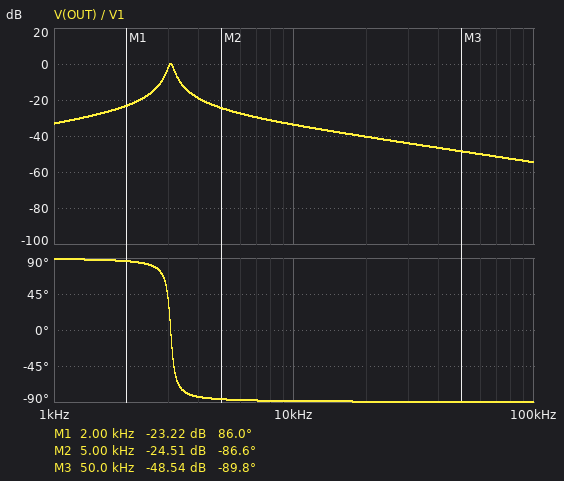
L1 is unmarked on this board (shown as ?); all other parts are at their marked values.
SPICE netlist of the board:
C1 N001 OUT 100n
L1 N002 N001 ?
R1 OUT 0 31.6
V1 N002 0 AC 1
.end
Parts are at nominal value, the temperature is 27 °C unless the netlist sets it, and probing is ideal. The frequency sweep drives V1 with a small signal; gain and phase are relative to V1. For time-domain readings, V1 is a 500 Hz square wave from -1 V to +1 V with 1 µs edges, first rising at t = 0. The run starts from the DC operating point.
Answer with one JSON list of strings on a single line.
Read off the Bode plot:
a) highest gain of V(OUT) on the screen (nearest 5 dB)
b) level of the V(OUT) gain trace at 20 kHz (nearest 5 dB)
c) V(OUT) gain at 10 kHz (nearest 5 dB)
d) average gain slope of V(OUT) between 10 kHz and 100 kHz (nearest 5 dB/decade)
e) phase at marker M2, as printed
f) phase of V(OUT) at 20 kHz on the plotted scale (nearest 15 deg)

["0 dB", "-40 dB", "-35 dB", "-20 dB/decade", "-86.6 deg", "-90 deg"]
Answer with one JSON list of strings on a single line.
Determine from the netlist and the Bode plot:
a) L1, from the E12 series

["27 mH"]
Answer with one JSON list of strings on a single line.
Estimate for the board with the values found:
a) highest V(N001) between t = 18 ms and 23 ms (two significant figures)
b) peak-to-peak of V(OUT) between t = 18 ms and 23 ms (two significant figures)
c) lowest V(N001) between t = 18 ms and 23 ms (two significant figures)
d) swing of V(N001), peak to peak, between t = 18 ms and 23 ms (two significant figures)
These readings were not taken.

["2.2 V", "150 mV", "-2.2 V", "4.4 V"]
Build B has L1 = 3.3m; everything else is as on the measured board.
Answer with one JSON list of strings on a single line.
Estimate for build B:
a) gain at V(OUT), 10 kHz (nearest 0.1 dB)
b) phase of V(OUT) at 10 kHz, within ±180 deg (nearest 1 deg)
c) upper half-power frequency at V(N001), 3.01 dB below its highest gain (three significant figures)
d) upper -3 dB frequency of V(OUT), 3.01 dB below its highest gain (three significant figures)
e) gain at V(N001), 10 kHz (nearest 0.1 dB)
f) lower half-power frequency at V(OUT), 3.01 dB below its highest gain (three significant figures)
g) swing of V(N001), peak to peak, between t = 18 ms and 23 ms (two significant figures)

["-5.2 dB", "-57 deg", "9.43 kHz", "9.56 kHz", "9.0 dB", "8.03 kHz", "5.1 V"]
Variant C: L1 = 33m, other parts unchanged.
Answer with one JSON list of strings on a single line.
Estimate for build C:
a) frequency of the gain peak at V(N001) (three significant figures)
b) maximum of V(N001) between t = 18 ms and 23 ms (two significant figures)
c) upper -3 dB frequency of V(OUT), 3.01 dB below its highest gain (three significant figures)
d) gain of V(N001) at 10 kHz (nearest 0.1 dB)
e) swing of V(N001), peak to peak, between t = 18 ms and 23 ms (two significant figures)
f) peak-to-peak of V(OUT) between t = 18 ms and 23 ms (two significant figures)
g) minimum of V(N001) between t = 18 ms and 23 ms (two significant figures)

["2.77 kHz", "2.5 V", "2.85 kHz", "-21.4 dB", "5.0 V", "170 mV", "-2.5 V"]
